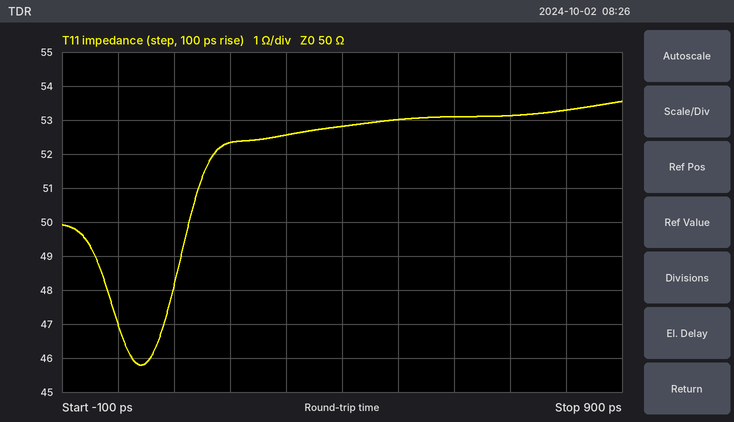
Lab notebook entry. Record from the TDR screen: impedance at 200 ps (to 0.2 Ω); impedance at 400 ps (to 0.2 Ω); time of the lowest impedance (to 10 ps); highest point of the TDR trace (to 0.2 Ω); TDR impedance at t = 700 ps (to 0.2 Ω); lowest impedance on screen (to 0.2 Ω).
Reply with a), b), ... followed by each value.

a) 52.4 Ω
b) 52.8 Ω
c) 40 ps
d) 53.6 Ω
e) 53.2 Ω
f) 45.8 Ω
